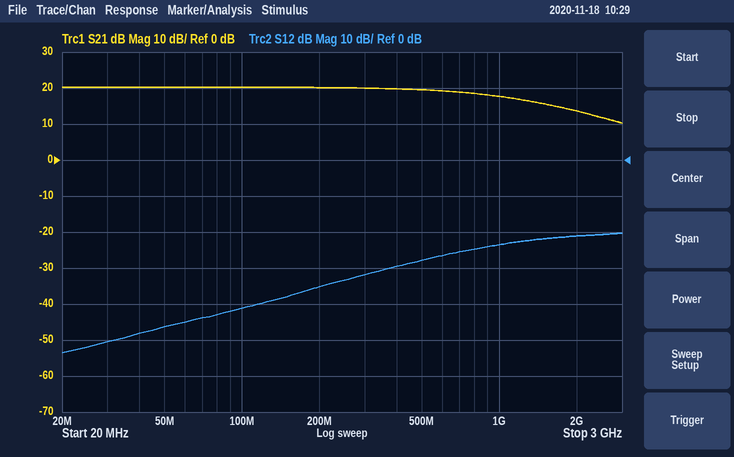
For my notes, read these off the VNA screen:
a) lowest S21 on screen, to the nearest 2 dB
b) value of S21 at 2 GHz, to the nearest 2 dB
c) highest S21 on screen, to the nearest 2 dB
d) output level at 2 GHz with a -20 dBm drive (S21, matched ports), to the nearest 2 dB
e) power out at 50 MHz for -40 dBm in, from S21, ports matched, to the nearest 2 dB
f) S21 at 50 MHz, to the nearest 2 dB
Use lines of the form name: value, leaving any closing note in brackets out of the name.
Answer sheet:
lowest S21 on screen, to the nearest 2 dB: 10 dB
value of S21 at 2 GHz, to the nearest 2 dB: 14 dB
highest S21 on screen, to the nearest 2 dB: 20 dB
output level at 2 GHz with a -20 dBm drive (S21, matched ports), to the nearest 2 dB: -6 dBm
power out at 50 MHz for -40 dBm in, from S21, ports matched, to the nearest 2 dB: -20 dBm
S21 at 50 MHz, to the nearest 2 dB: 20 dB
